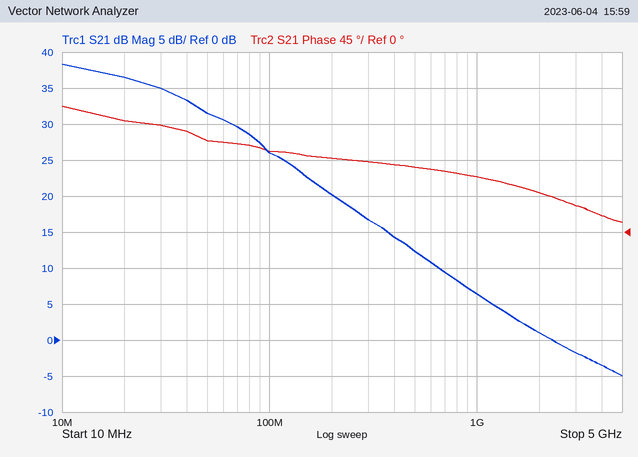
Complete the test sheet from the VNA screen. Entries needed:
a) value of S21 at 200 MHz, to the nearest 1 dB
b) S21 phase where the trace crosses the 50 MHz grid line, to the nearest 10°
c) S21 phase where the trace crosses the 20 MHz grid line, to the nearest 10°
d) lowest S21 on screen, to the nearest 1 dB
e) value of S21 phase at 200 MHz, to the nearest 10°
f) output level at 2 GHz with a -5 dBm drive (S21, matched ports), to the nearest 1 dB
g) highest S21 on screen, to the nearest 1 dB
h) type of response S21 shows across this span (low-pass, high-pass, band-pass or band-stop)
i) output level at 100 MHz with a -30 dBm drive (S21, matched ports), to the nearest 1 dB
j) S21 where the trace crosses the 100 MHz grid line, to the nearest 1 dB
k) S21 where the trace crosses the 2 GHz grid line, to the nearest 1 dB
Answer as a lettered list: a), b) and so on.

a) 20 dB
b) 110°
c) 140°
d) -5 dB
e) 90°
f) -4 dBm
g) 38 dB
h) low-pass
i) -4 dBm
j) 26 dB
k) 1 dB
